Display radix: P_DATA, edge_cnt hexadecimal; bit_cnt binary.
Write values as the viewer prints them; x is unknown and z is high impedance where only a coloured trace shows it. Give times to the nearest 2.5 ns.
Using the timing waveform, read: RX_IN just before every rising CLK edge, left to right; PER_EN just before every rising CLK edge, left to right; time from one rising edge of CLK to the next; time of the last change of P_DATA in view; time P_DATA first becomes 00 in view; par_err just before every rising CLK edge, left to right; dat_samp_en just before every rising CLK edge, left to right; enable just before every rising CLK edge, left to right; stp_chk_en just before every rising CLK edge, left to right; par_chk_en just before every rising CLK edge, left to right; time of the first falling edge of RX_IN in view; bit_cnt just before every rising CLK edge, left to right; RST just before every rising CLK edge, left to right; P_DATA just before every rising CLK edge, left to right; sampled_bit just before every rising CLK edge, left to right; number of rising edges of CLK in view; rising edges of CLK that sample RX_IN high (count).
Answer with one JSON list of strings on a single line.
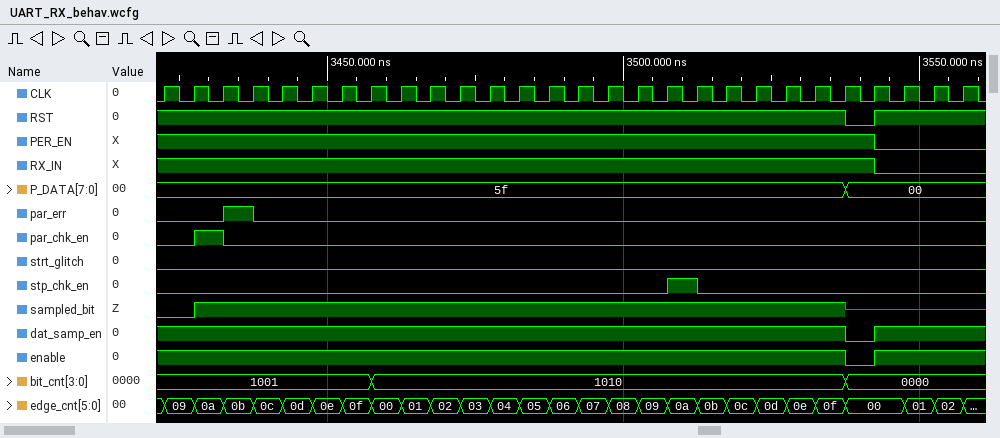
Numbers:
["1 1 1 1 1 1 1 1 1 1 1 1 1 1 1 1 1 1 1 1 1 1 1 1 1 0 0 0", "1 1 1 1 1 1 1 1 1 1 1 1 1 1 1 1 1 1 1 1 1 1 1 1 1 0 0 0", "5 ns", "3537.5 ns", "3537.5 ns", "0 0 0 1 0 0 0 0 0 0 0 0 0 0 0 0 0 0 0 0 0 0 0 0 0 0 0 0", "1 1 1 1 1 1 1 1 1 1 1 1 1 1 1 1 1 1 1 1 1 1 1 1 0 1 1 1", "1 1 1 1 1 1 1 1 1 1 1 1 1 1 1 1 1 1 1 1 1 1 1 1 0 1 1 1", "0 0 0 0 0 0 0 0 0 0 0 0 0 0 0 0 0 0 1 0 0 0 0 0 0 0 0 0", "0 0 1 0 0 0 0 0 0 0 0 0 0 0 0 0 0 0 0 0 0 0 0 0 0 0 0 0", "3542.5 ns", "1001, 1001, 1001, 1001, 1001, 1001, 1001, 1001, 1010, 1010, 1010, 1010, 1010, 1010, 1010, 1010, 1010, 1010, 1010, 1010, 1010, 1010, 1010, 1010, 0000, 0000, 0000, 0000", "1 1 1 1 1 1 1 1 1 1 1 1 1 1 1 1 1 1 1 1 1 1 1 1 0 1 1 1", "5f, 5f, 5f, 5f, 5f, 5f, 5f, 5f, 5f, 5f, 5f, 5f, 5f, 5f, 5f, 5f, 5f, 5f, 5f, 5f, 5f, 5f, 5f, 5f, 00, 00, 00, 00", "0 0 1 1 1 1 1 1 1 1 1 1 1 1 1 1 1 1 1 1 1 1 1 1 z z z z", "28", "25"]
